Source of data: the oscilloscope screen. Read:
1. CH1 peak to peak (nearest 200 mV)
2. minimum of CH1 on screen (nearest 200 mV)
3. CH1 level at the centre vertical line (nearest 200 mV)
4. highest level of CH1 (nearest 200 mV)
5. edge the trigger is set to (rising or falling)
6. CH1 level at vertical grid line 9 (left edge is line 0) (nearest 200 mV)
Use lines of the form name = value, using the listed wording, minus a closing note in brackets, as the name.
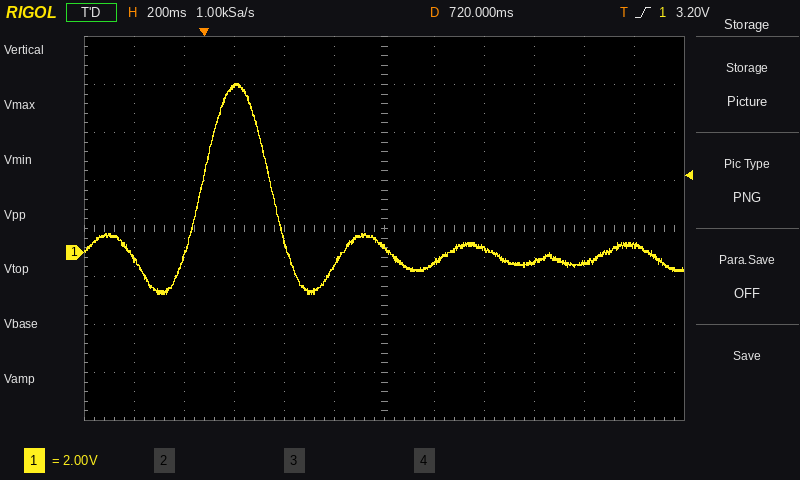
CH1 peak to peak = 8.8 V
minimum of CH1 on screen = -1.8 V
CH1 level at the centre vertical line = 200 mV
highest level of CH1 = 7.0 V
edge the trigger is set to = rising
CH1 level at vertical grid line 9 (left edge is line 0) = -400 mV
